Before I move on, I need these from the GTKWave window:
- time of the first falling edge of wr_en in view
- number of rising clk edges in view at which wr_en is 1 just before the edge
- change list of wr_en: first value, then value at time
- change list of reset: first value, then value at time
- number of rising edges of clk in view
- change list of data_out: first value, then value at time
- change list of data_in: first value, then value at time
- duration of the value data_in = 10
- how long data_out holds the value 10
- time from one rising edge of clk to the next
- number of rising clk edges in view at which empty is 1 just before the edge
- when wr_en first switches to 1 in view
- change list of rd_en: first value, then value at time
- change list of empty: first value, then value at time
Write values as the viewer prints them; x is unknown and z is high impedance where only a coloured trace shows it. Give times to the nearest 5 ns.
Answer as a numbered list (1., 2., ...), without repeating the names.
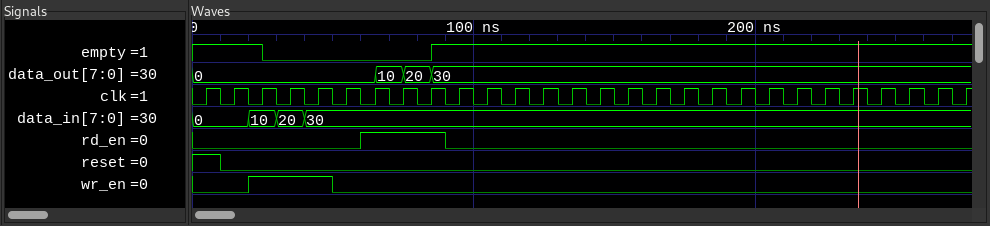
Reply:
1. 50 ns
2. 3
3. 0, 1 at 20 ns, 0 at 50 ns
4. 1, 0 at 10 ns
5. 28
6. 0, 10 at 65 ns, 20 at 75 ns, 30 at 85 ns
7. 0, 10 at 20 ns, 20 at 30 ns, 30 at 40 ns
8. 10 ns
9. 10 ns
10. 10 ns
11. 22
12. 20 ns
13. 0, 1 at 60 ns, 0 at 90 ns
14. 1, 0 at 25 ns, 1 at 85 ns
